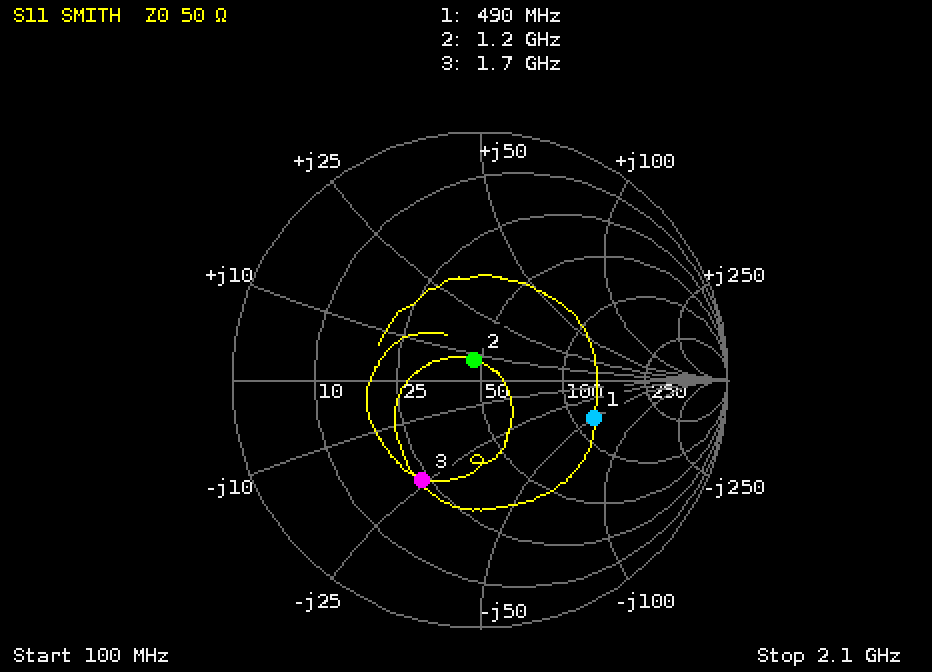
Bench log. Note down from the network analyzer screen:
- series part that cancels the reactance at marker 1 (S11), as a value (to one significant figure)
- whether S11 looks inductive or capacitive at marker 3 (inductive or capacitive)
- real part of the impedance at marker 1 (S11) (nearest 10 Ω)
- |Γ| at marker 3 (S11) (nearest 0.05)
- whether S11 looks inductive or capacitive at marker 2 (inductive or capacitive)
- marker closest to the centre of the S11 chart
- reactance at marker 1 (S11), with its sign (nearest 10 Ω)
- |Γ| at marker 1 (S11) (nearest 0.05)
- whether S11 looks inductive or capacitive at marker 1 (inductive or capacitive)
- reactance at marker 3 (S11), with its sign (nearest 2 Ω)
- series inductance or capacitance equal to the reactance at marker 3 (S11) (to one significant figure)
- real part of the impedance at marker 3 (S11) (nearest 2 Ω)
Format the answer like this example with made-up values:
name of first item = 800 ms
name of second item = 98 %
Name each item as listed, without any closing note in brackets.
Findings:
series part that cancels the reactance at marker 1 (S11), as a value = 20 nH
whether S11 looks inductive or capacitive at marker 3 = capacitive
real part of the impedance at marker 1 (S11) = 120 Ω
|Γ| at marker 3 (S11) = 0.45
whether S11 looks inductive or capacitive at marker 2 = inductive
marker closest to the centre of the S11 chart = marker 2
reactance at marker 1 (S11), with its sign = -50 Ω
|Γ| at marker 1 (S11) = 0.50
whether S11 looks inductive or capacitive at marker 1 = capacitive
reactance at marker 3 (S11), with its sign = -24 Ω
series inductance or capacitance equal to the reactance at marker 3 (S11) = 4 pF
real part of the impedance at marker 3 (S11) = 24 Ω
